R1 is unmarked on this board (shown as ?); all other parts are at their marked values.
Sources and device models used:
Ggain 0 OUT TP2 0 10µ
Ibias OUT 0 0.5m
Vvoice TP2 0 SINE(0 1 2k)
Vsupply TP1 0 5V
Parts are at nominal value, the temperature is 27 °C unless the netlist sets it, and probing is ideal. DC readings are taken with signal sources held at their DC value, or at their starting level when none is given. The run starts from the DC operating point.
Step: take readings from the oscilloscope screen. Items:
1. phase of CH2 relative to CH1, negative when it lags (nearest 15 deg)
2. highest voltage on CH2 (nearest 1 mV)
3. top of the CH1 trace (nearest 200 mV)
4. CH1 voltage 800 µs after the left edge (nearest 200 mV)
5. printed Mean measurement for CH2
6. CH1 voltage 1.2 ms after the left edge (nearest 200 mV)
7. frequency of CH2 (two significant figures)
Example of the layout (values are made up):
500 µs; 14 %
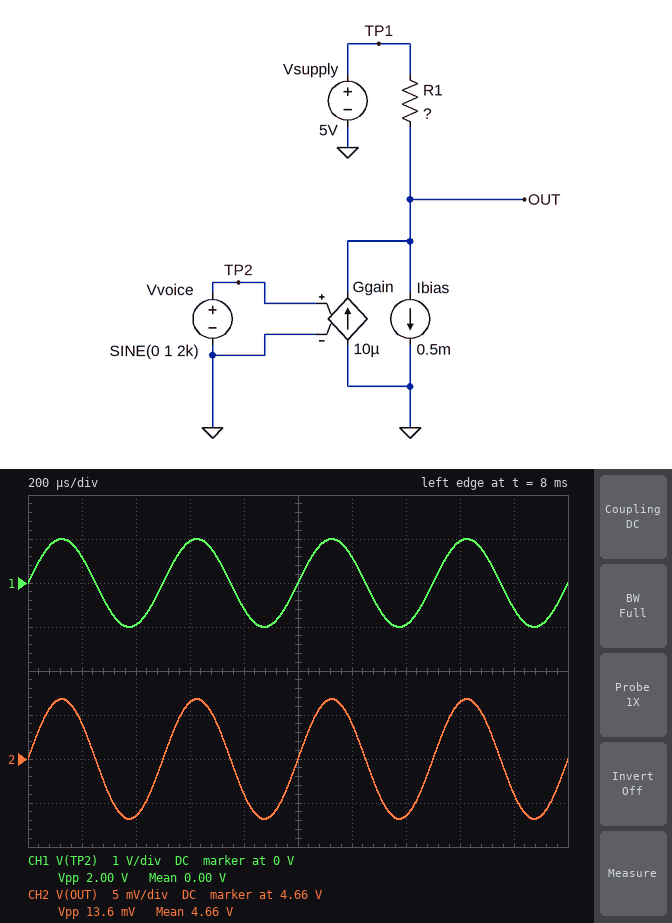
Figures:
0 deg; 4.667 V; 1.0 V; -600 mV; 4.66 V; 600 mV; 2.0 kHz
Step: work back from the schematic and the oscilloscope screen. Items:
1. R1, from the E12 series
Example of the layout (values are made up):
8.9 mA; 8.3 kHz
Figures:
680 Ω
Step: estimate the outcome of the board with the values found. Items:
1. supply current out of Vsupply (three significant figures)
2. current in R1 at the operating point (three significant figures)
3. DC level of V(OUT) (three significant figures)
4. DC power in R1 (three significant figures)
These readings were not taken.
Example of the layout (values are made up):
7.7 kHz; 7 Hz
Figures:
500 µA; 500 µA; 4.66 V; 170 µW
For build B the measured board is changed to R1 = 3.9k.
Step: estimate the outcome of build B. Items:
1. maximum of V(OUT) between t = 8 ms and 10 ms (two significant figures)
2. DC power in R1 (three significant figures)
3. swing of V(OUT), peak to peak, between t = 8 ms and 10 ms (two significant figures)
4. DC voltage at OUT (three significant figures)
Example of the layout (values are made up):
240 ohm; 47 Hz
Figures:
3.1 V; 975 µW; 78 mV; 3.05 V
